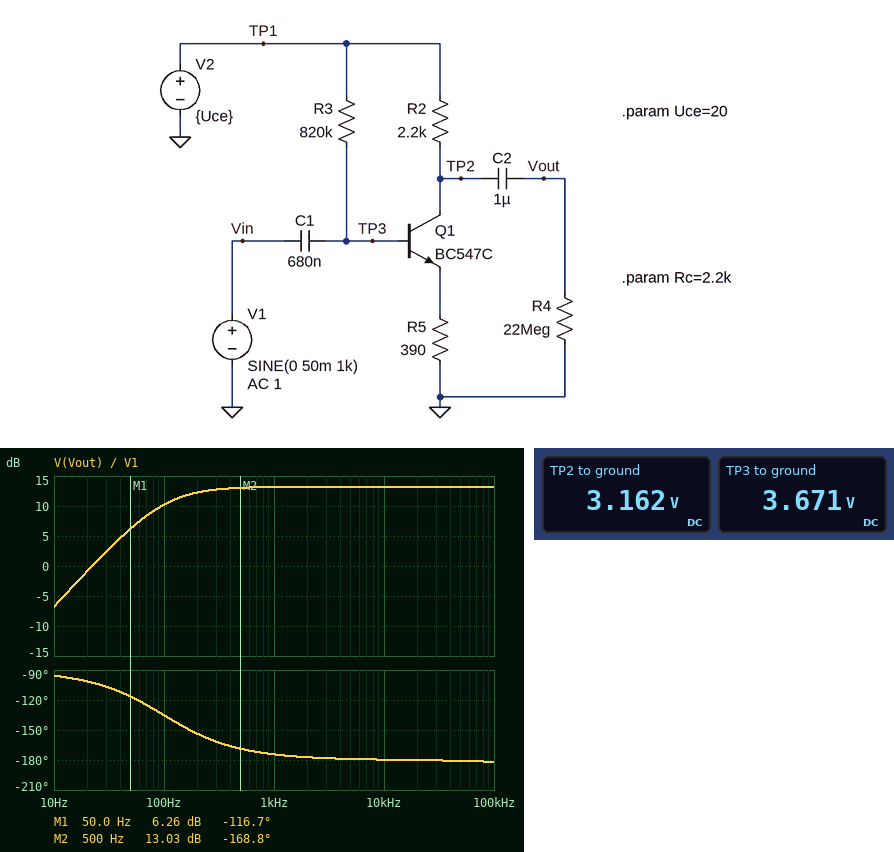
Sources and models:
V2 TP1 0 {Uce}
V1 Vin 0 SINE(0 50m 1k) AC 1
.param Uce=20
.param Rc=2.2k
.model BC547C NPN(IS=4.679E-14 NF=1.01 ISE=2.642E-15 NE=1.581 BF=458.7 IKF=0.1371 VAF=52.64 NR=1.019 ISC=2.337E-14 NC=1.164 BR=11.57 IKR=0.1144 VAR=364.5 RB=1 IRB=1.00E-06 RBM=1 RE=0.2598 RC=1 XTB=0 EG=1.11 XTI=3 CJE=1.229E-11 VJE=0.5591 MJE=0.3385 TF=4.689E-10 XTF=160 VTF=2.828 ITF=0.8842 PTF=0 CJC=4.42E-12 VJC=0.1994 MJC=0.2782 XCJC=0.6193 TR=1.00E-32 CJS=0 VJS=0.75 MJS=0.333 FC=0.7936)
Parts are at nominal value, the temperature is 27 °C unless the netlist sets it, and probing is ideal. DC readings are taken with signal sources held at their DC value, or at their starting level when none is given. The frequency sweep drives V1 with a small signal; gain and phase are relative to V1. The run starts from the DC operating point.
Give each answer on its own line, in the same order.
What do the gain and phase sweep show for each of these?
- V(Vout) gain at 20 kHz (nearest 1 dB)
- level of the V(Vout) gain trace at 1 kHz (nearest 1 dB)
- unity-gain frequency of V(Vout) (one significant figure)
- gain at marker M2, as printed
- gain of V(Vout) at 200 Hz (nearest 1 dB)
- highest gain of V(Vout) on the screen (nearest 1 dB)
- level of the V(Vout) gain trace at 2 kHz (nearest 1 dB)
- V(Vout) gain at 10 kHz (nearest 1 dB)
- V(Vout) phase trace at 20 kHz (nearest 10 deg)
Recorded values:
13 dB
13 dB
20 Hz
13.03 dB
12 dB
13 dB
13 dB
13 dB
-180 deg
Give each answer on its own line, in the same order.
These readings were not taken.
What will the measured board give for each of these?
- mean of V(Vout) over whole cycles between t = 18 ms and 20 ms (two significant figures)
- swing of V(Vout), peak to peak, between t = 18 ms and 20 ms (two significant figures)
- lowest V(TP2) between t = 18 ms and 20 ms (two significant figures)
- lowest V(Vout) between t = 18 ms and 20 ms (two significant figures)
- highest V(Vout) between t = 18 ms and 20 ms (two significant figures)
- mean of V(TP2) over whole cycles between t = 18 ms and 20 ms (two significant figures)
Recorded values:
200 mV
520 mV
3.1 V
-42 mV
480 mV
3.4 V
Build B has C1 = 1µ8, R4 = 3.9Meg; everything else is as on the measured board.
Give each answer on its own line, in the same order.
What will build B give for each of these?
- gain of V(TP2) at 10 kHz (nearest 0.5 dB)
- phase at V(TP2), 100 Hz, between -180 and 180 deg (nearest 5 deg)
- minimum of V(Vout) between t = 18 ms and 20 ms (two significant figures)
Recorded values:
13.0 dB
-160 deg
-44 mV
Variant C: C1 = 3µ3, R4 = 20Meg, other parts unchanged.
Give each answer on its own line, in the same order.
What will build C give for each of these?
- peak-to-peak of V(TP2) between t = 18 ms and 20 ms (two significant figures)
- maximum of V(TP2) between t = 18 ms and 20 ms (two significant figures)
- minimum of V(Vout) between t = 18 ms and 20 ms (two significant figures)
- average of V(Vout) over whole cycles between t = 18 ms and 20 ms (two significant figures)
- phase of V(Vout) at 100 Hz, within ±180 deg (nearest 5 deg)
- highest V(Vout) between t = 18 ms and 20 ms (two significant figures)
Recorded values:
510 mV
3.6 V
-47 mV
190 mV
-170 deg
460 mV
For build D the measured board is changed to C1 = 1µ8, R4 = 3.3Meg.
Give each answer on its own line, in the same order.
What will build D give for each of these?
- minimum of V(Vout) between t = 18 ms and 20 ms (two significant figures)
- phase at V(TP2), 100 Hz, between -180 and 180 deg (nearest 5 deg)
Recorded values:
-44 mV
-160 deg
